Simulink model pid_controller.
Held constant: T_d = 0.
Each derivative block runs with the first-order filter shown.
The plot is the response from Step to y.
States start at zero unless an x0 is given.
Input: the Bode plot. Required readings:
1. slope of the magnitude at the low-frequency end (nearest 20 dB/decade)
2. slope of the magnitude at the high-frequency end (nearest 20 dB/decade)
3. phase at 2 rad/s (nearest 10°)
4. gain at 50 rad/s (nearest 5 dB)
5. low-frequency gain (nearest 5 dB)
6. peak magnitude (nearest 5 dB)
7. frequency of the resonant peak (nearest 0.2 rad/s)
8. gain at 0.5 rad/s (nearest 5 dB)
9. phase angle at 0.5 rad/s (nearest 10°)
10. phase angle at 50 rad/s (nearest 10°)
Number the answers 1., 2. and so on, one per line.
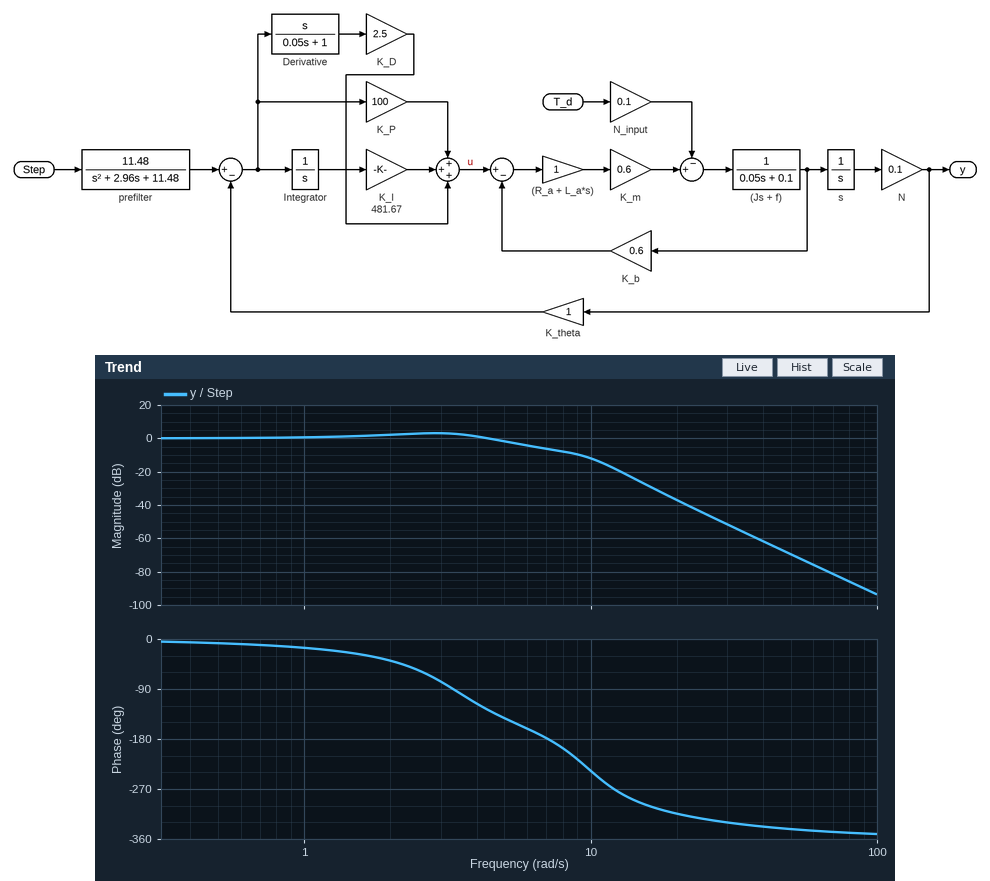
1. 0 dB/decade
2. -80 dB/decade
3. -40°
4. -70 dB
5. 0 dB
6. 5 dB
7. 2.8 rad/s
8. 0 dB
9. -10°
10. -340°
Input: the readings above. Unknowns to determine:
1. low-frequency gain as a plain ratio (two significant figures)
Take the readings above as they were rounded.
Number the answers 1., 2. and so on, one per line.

1. 1.0
